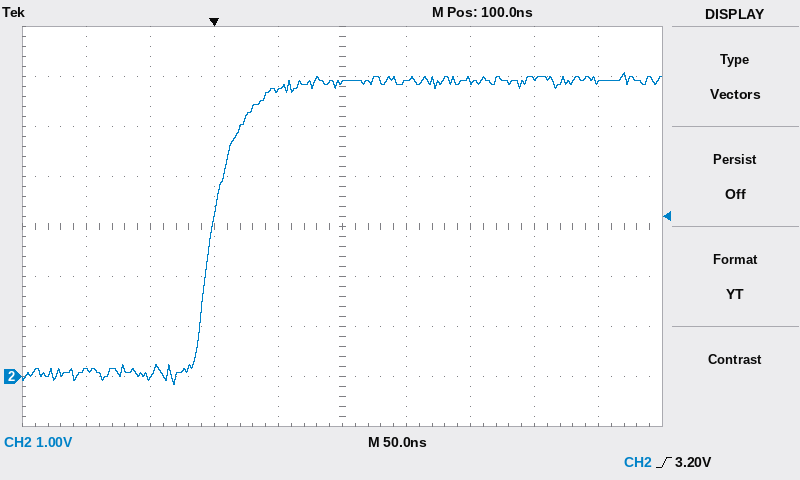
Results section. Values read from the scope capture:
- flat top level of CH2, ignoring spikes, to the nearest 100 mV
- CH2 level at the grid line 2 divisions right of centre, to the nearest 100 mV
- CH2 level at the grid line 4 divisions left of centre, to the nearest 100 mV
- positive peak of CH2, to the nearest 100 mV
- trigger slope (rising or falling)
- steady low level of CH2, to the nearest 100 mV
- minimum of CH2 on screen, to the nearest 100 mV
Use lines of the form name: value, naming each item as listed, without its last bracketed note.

flat top level of CH2, ignoring spikes, to the nearest 100 mV: 5.9 V
CH2 level at the grid line 2 divisions right of centre, to the nearest 100 mV: 5.9 V
CH2 level at the grid line 4 divisions left of centre, to the nearest 100 mV: 100 mV
positive peak of CH2, to the nearest 100 mV: 6.1 V
trigger slope: rising
steady low level of CH2, to the nearest 100 mV: 100 mV
minimum of CH2 on screen, to the nearest 100 mV: -200 mV
